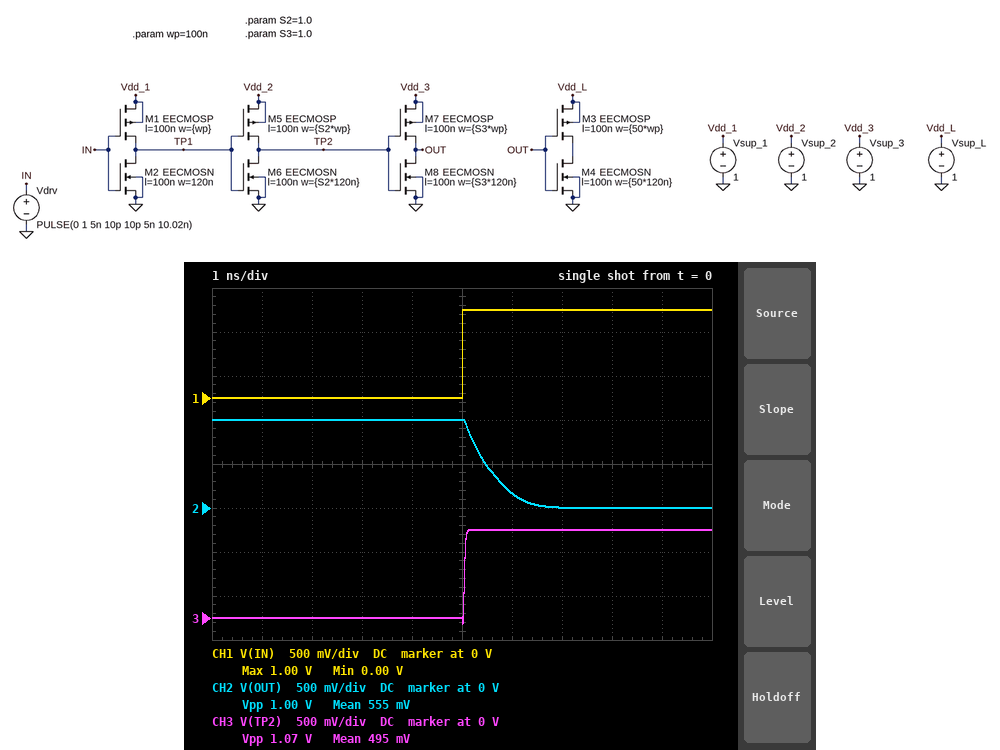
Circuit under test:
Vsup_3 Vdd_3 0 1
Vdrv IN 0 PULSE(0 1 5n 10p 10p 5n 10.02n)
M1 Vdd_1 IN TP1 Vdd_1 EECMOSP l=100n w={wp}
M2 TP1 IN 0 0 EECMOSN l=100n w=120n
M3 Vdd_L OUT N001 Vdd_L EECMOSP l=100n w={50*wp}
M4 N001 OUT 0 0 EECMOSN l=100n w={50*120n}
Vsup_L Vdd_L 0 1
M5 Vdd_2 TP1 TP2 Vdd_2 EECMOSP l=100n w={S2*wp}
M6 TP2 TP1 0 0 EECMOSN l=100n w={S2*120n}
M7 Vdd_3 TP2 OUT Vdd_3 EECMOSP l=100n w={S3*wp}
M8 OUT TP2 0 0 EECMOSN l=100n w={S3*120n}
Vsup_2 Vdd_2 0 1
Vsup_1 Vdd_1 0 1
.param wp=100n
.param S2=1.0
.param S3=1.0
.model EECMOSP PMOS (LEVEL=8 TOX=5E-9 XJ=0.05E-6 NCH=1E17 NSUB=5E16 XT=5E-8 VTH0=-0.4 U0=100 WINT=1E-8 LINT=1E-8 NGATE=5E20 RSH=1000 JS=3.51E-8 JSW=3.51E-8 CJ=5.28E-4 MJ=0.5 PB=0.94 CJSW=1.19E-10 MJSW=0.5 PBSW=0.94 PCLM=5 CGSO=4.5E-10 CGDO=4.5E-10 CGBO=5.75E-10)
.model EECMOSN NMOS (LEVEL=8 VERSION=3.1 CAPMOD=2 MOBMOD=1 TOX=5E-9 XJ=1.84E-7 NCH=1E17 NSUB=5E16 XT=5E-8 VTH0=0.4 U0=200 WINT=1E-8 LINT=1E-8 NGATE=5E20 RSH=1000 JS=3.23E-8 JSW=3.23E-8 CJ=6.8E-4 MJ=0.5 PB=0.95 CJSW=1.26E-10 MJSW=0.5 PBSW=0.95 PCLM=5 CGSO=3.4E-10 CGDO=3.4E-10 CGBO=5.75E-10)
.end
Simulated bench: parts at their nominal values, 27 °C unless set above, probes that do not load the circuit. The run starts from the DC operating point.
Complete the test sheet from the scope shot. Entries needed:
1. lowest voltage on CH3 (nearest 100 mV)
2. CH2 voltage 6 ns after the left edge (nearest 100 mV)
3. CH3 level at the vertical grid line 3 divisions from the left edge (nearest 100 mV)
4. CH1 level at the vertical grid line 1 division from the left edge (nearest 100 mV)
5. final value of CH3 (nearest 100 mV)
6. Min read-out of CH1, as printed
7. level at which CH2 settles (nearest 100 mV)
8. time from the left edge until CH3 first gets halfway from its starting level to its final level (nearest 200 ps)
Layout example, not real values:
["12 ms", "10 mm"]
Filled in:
["-100 mV", "200 mV", "0 V", "0 V", "1.0 V", "0.00 V", "0 V", "5.0 ns"]
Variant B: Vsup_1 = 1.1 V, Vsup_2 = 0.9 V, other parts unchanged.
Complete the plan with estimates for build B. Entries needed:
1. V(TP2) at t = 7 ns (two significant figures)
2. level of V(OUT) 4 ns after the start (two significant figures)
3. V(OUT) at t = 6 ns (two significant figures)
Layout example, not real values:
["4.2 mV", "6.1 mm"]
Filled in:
["900 mV", "1.0 V", "230 mV"]
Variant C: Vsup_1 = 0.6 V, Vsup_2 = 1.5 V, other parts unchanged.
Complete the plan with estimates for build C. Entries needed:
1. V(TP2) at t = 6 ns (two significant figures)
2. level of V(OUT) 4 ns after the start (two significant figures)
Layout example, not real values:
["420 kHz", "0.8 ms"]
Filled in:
["1.5 V", "43 mV"]
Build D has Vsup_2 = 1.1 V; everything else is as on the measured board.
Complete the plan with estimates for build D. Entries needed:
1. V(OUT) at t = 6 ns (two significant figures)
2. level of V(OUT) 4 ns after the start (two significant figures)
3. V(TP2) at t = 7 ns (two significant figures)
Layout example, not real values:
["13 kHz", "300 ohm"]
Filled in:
["120 mV", "1.0 V", "1.1 V"]
